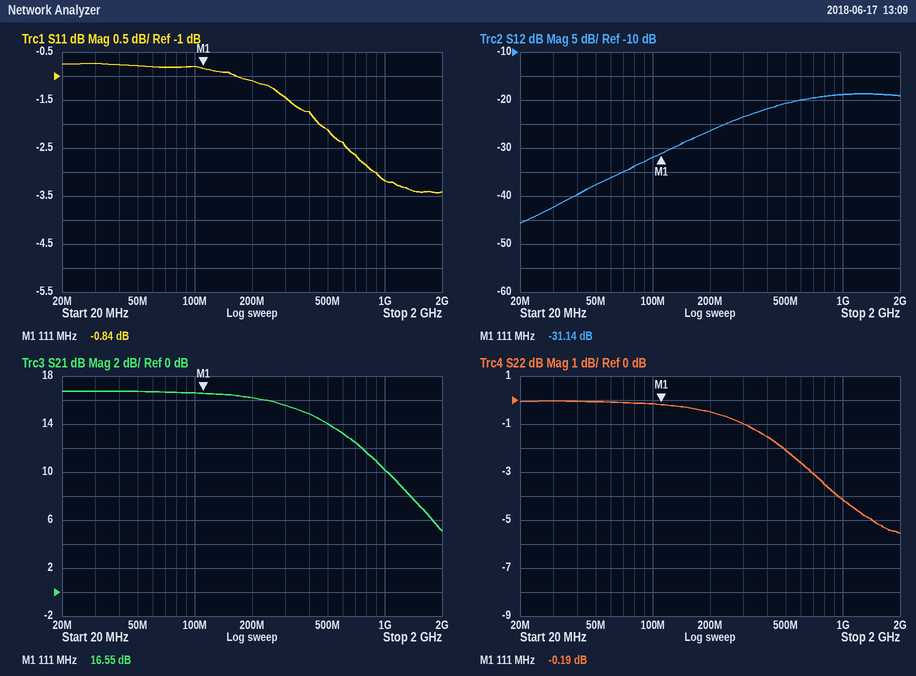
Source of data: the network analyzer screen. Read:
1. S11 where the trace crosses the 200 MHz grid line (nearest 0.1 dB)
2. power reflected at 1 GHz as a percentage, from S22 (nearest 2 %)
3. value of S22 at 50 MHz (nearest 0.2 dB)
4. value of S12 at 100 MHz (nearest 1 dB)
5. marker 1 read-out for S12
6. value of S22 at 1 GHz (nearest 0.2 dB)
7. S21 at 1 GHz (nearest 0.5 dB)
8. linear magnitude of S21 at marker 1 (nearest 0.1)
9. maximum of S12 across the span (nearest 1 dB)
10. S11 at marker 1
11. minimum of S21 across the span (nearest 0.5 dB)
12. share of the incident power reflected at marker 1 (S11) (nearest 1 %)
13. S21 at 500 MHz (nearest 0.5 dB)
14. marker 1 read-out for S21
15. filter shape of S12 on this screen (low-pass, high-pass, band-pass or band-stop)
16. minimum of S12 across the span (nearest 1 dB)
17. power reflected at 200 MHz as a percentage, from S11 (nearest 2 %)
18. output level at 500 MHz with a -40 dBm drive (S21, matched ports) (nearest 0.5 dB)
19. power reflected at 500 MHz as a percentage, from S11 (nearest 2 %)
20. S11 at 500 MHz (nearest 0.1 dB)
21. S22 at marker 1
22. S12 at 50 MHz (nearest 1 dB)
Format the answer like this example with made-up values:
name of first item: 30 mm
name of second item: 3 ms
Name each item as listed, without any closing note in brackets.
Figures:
S11 where the trace crosses the 200 MHz grid line: -1.1 dB
power reflected at 1 GHz as a percentage, from S22: 38 %
value of S22 at 50 MHz: 0.0 dB
value of S12 at 100 MHz: -32 dB
marker 1 read-out for S12: -31.14 dB
value of S22 at 1 GHz: -4.2 dB
S21 at 1 GHz: 10.0 dB
linear magnitude of S21 at marker 1: 6.7
maximum of S12 across the span: -19 dB
S11 at marker 1: -0.84 dB
minimum of S21 across the span: 5.0 dB
share of the incident power reflected at marker 1 (S11): 82 %
S21 at 500 MHz: 14.0 dB
marker 1 read-out for S21: 16.55 dB
filter shape of S12 on this screen: high-pass
minimum of S12 across the span: -46 dB
power reflected at 200 MHz as a percentage, from S11: 78 %
output level at 500 MHz with a -40 dBm drive (S21, matched ports): -26.0 dBm
power reflected at 500 MHz as a percentage, from S11: 62 %
S11 at 500 MHz: -2.1 dB
S22 at marker 1: -0.19 dB
S12 at 50 MHz: -38 dB
